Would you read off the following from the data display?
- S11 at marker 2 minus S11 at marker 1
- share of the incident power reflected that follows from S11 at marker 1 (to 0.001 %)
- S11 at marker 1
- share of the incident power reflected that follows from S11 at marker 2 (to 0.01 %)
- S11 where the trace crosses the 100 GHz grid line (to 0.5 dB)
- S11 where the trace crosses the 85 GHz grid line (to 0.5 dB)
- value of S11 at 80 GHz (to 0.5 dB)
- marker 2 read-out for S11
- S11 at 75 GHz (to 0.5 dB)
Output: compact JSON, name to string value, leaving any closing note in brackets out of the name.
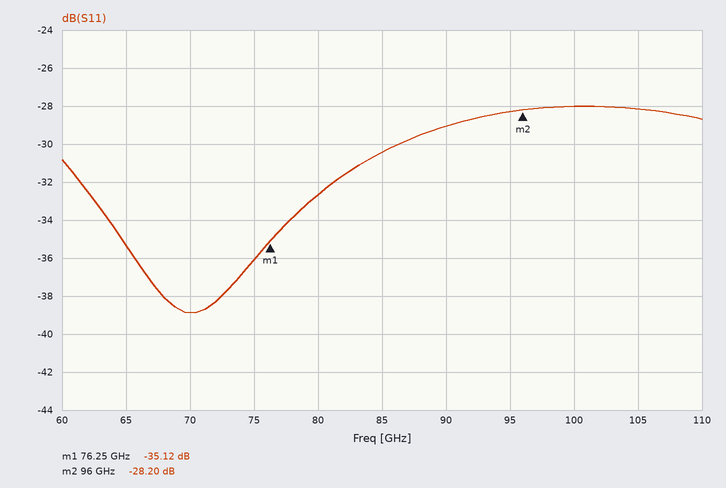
{"S11 at marker 2 minus S11 at marker 1": "6.92 dB", "share of the incident power reflected that follows from S11 at marker 1": "0.031 %", "S11 at marker 1": "-35.12 dB", "share of the incident power reflected that follows from S11 at marker 2": "0.15 %", "S11 where the trace crosses the 100 GHz grid line": "-28.0 dB", "S11 where the trace crosses the 85 GHz grid line": "-30.5 dB", "value of S11 at 80 GHz": "-32.5 dB", "marker 2 read-out for S11": "-28.20 dB", "S11 at 75 GHz": "-36.0 dB"}
